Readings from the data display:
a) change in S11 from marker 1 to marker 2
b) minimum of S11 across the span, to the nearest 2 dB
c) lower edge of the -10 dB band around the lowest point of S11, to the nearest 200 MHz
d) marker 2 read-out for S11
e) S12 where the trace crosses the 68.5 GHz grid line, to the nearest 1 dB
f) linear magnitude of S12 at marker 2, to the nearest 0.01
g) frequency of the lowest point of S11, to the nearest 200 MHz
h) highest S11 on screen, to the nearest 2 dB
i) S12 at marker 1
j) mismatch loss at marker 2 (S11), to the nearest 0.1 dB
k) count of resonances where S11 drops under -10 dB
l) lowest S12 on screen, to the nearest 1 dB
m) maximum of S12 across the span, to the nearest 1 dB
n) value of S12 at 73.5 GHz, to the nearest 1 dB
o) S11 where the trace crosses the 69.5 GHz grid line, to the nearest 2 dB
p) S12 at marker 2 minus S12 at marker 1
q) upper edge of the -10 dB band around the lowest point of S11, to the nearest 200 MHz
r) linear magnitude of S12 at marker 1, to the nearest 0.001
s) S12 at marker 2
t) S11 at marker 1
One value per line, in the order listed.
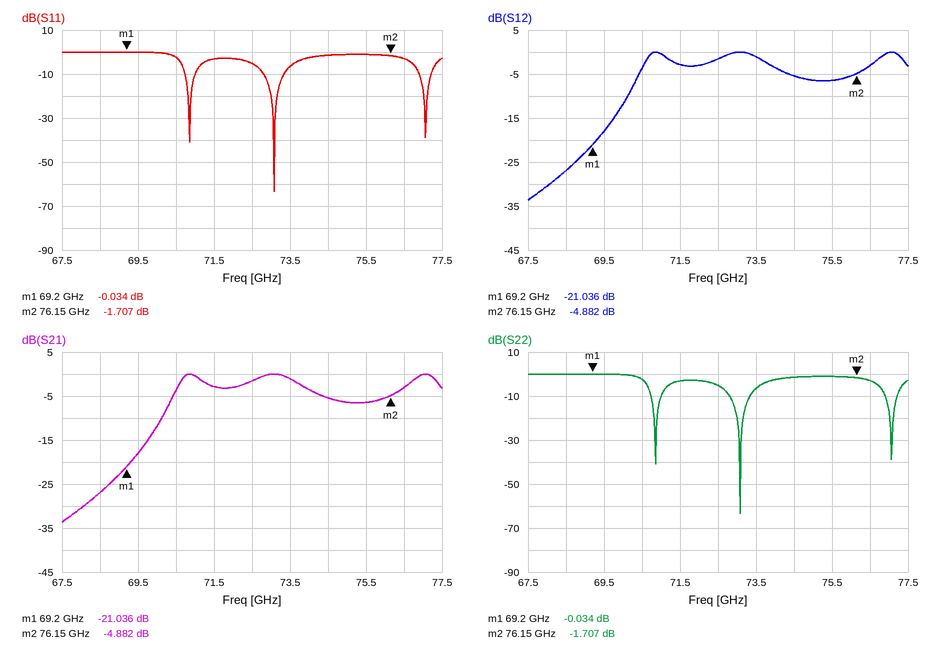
-1.673 dB
-64 dB
72.8 GHz
-1.707 dB
-27 dB
0.57
73.0 GHz
0 dB
-21.036 dB
4.9 dB
3
-34 dB
0 dB
-1 dB
0 dB
16.154 dB
73.4 GHz
0.089
-4.882 dB
-0.034 dB
